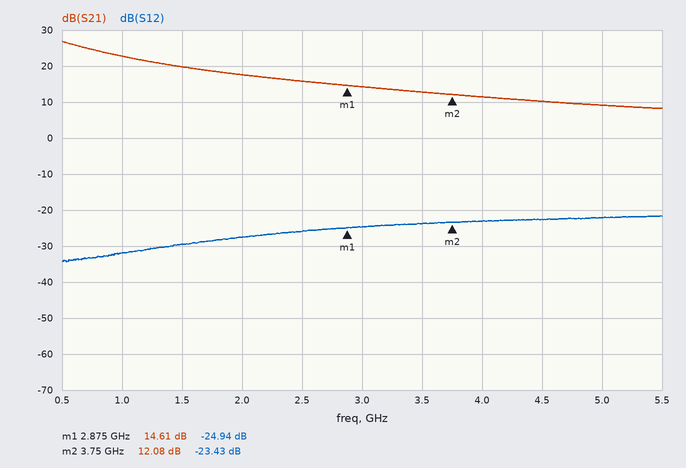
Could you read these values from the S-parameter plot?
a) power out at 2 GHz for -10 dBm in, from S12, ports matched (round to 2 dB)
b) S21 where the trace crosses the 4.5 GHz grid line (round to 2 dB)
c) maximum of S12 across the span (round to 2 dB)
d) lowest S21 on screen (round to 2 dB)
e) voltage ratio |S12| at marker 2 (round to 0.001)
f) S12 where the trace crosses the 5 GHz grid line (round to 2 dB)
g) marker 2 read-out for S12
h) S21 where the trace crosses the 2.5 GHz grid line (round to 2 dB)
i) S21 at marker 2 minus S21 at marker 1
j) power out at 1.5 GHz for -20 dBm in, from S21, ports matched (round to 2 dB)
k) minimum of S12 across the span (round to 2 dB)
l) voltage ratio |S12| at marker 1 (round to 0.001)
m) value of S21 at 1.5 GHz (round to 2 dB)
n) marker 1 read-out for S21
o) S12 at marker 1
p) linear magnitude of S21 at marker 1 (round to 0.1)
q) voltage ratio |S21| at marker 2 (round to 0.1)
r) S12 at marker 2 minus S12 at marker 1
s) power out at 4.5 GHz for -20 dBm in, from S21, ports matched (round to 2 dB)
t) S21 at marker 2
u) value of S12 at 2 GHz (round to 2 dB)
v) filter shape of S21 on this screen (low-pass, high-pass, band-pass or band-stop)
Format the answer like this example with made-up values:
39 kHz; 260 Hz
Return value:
-38 dBm; 10 dB; -22 dB; 8 dB; 0.067; -22 dB; -23.43 dB; 16 dB; -2.53 dB; 0 dBm; -34 dB; 0.057; 20 dB; 14.61 dB; -24.94 dB; 5.4; 4.0; 1.51 dB; -10 dBm; 12.08 dB; -28 dB; low-pass
